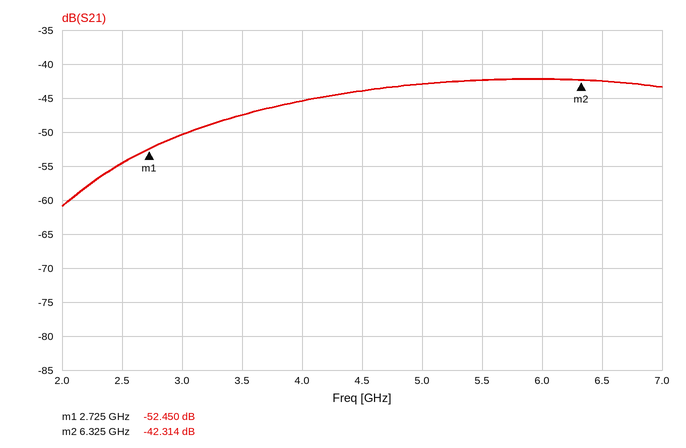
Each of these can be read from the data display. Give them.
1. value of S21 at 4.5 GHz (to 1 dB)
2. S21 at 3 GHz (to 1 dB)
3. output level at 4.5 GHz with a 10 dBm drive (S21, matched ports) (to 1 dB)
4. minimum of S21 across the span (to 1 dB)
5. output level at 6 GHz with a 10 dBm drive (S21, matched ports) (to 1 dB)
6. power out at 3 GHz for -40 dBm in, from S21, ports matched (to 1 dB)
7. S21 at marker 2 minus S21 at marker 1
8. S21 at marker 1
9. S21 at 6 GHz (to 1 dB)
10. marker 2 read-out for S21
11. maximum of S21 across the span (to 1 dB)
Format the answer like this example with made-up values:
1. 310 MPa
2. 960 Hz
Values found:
1. -44 dB
2. -50 dB
3. -34 dBm
4. -61 dB
5. -32 dBm
6. -90 dBm
7. 10.136 dB
8. -52.450 dB
9. -42 dB
10. -42.314 dB
11. -42 dB
